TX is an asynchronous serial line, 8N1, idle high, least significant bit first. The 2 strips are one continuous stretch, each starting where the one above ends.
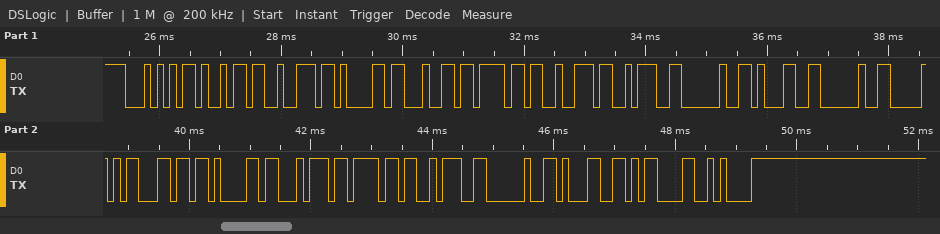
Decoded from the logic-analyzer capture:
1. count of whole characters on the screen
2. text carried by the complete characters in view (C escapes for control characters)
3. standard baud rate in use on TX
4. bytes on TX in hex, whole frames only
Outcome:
21
"Tirador: 1 Plato: 1\r\n"
9600 baud
54 69 72 61 64 6F 72 3A 20 31 20 50 6C 61 74 6F 3A 20 31 0D 0A
